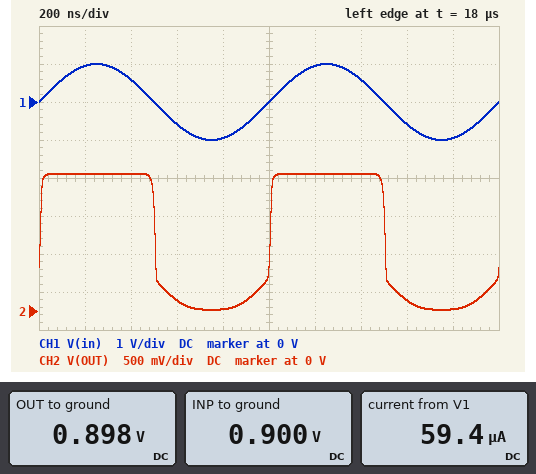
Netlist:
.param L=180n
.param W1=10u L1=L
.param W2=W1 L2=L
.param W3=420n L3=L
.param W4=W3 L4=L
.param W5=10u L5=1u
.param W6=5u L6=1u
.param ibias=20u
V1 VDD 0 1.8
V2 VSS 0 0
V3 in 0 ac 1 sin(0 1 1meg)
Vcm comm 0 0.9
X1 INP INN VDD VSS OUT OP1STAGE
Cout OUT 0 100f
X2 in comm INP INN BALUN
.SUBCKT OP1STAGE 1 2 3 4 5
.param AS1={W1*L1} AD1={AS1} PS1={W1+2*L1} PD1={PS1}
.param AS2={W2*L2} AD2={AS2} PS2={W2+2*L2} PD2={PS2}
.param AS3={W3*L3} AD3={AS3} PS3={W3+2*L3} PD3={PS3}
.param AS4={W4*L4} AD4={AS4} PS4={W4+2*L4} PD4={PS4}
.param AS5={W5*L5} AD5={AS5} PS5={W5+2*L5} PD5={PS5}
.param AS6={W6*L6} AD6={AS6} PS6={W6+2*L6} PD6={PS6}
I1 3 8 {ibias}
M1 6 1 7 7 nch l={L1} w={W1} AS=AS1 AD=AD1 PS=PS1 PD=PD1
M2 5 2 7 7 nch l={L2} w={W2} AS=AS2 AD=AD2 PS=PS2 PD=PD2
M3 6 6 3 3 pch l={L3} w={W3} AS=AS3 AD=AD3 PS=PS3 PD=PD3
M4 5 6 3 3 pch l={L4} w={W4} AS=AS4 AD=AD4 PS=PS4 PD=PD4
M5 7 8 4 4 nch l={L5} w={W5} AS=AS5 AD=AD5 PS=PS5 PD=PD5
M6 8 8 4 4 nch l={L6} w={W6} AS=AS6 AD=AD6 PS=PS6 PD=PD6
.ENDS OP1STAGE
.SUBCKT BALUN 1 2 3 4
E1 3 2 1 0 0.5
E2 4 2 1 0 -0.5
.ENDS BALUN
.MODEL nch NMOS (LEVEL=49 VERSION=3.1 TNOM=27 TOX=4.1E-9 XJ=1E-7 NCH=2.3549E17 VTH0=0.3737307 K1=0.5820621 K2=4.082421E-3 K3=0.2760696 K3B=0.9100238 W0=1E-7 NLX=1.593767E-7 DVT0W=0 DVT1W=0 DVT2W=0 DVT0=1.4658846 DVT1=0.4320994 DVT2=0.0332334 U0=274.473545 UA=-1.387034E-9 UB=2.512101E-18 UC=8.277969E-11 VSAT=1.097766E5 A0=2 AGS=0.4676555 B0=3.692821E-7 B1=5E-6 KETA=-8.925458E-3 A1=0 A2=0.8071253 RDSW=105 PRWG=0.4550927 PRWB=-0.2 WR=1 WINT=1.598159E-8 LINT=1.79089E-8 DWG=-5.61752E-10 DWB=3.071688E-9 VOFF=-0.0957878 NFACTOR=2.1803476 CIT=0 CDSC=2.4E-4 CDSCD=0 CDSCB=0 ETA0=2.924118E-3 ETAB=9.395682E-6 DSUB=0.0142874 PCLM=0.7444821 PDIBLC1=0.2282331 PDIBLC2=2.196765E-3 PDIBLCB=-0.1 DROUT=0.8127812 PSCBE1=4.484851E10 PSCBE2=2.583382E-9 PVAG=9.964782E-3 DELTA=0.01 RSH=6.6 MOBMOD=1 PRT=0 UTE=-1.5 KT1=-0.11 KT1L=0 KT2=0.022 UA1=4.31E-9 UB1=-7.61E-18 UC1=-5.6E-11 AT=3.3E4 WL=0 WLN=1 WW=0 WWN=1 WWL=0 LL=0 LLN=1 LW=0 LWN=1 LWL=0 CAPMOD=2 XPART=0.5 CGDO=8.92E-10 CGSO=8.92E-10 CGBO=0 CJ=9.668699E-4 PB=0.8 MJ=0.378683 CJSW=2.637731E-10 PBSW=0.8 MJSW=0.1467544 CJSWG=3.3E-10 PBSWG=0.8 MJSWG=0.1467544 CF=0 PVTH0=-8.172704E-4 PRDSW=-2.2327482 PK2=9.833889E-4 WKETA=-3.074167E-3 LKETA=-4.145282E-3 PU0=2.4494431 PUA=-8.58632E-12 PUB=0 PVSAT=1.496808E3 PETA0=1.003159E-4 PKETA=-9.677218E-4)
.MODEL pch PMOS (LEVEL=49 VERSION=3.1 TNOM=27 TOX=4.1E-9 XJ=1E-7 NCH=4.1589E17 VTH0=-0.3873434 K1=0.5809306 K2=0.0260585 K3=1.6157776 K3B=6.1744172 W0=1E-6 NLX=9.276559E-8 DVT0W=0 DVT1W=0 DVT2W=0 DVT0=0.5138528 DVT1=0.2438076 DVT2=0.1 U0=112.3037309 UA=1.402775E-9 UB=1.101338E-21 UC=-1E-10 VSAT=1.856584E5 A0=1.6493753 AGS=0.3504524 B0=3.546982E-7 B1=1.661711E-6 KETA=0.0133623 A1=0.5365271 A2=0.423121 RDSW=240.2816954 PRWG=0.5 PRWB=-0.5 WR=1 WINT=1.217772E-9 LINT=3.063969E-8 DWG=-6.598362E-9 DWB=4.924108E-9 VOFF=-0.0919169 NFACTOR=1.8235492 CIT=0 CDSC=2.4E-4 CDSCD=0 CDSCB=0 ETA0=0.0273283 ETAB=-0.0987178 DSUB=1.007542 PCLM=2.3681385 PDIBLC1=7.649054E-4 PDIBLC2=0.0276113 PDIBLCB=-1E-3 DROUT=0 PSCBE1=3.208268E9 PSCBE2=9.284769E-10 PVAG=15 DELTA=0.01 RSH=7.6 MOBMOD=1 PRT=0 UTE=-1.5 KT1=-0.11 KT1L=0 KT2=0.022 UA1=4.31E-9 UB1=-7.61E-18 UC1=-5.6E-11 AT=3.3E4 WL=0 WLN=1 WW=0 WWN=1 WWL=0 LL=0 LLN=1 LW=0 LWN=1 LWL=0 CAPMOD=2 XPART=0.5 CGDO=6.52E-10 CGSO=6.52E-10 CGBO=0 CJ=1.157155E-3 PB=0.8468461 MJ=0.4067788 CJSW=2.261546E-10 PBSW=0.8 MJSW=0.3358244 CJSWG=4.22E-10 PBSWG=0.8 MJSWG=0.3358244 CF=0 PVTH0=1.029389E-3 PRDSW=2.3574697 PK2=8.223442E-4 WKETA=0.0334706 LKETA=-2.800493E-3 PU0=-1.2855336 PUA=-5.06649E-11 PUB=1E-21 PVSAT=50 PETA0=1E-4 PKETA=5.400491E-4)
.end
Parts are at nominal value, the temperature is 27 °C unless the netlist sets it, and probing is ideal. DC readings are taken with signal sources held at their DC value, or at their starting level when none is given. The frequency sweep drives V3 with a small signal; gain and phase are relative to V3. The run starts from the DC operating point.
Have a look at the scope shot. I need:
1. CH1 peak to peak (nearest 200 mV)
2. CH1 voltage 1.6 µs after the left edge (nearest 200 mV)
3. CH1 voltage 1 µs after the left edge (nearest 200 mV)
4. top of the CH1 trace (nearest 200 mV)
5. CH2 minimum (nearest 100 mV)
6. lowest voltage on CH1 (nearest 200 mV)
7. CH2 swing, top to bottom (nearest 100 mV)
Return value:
2.0 V
-600 mV
0 V
1.0 V
0 V
-1.0 V
1.8 V
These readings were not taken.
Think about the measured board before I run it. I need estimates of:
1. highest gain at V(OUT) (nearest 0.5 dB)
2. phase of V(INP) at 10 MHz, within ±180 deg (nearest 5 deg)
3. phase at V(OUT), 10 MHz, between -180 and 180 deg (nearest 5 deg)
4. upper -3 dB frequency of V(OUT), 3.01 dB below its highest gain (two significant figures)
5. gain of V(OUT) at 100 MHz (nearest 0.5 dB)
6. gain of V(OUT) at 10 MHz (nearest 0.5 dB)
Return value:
28.0 dB
0 deg
-25 deg
21 MHz
14.5 dB
27.0 dB
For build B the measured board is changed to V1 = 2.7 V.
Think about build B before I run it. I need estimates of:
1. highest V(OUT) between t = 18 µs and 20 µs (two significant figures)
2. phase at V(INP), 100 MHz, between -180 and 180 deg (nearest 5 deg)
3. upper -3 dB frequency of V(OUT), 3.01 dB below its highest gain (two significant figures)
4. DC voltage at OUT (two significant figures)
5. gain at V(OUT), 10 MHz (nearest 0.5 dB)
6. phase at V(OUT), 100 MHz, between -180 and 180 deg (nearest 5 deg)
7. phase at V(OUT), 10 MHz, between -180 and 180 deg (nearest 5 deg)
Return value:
2.7 V
0 deg
18 MHz
1.8 V
28.5 dB
-85 deg
-30 deg
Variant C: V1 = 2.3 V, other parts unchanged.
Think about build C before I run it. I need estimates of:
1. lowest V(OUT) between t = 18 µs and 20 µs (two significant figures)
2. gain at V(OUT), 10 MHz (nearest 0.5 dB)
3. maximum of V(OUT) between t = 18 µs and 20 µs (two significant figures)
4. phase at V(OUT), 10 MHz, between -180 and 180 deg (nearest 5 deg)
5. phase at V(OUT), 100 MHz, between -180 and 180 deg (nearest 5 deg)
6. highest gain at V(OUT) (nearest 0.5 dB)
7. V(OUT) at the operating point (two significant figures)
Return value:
19 mV
28.0 dB
2.3 V
-30 deg
-85 deg
29.0 dB
1.4 V
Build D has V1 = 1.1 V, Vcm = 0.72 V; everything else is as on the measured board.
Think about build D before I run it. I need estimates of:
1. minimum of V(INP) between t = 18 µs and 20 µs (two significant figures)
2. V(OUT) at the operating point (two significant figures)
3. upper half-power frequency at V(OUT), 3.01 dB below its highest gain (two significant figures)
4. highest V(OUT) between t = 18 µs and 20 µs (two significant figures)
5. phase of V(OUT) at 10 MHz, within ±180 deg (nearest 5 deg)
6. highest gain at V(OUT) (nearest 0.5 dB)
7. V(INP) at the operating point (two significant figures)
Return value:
220 mV
210 mV
150 MHz
1.1 V
-5 deg
-6.5 dB
720 mV
